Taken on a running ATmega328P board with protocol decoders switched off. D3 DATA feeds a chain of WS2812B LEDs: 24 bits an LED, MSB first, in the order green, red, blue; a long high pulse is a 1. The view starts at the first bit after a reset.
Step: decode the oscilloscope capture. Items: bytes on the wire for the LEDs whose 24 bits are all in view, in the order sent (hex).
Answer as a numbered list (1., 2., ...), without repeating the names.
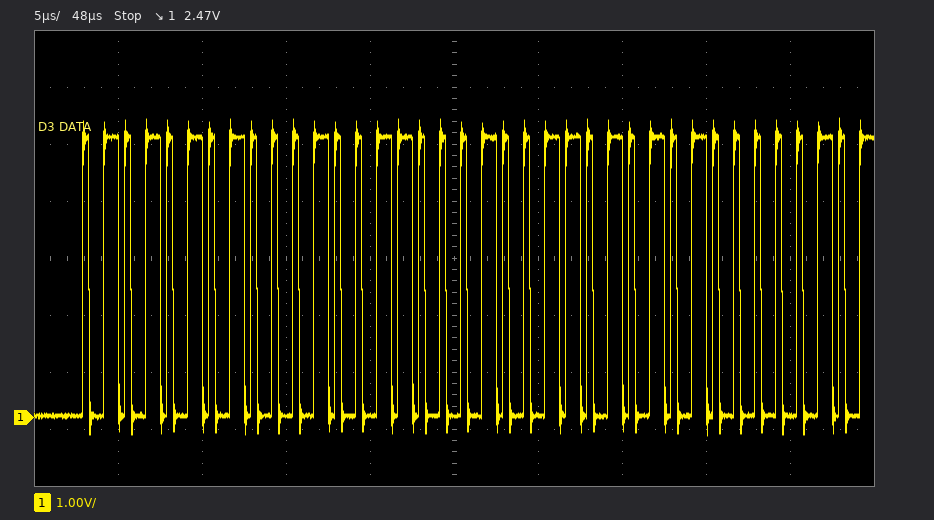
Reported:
1. 55 13 13
